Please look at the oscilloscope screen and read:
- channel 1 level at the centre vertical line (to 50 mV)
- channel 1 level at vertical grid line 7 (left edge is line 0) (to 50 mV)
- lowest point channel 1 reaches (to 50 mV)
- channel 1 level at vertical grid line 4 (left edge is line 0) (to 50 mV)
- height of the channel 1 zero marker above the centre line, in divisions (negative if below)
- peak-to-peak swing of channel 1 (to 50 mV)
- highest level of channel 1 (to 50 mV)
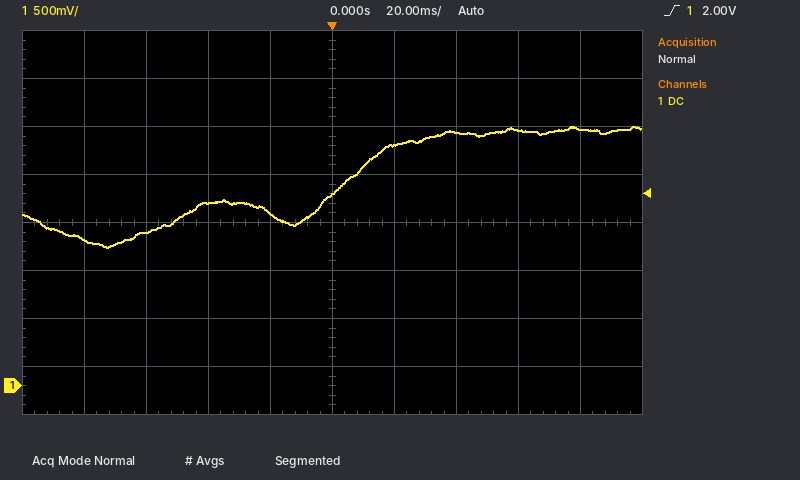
2.00 V
2.65 V
1.45 V
1.80 V
-3.4 div
1.25 V
2.70 V
